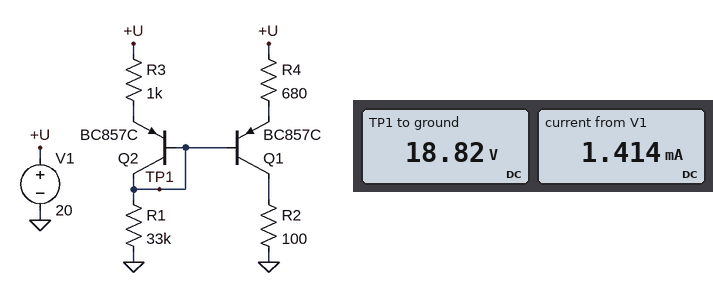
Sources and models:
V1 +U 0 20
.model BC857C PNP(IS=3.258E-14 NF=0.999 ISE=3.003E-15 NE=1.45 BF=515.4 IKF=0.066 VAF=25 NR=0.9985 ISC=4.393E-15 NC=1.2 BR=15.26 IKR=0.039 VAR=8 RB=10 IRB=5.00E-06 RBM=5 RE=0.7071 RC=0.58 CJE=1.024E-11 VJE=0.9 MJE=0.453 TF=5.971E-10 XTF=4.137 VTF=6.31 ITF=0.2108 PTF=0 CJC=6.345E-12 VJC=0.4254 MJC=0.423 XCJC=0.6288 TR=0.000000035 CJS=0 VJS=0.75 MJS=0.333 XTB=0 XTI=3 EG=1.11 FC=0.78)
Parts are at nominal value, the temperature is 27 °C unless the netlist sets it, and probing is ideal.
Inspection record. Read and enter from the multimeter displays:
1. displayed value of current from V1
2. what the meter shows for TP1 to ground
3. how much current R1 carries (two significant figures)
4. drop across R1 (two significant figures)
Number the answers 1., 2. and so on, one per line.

1. 1.414 mA
2. 18.82 V
3. 570 µA
4. 19 V
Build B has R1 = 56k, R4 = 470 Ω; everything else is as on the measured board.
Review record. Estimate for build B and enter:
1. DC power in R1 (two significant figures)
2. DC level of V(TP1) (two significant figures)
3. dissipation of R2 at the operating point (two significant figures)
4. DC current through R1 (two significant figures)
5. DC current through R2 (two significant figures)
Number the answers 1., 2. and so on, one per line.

1. 6.5 mW
2. 19 V
3. 51 µW
4. 340 µA
5. 710 µA
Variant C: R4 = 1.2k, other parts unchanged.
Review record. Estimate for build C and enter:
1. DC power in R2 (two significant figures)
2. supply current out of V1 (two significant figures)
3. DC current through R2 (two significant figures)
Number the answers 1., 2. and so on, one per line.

1. 24 µW
2. 1.1 mA
3. 490 µA
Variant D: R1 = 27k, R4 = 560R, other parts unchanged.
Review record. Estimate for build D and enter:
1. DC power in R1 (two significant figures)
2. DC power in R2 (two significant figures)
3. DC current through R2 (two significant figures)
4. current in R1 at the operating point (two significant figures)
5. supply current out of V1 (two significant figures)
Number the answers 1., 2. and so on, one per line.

1. 13 mW
2. 150 µW
3. 1.2 mA
4. 690 µA
5. 1.9 mA
